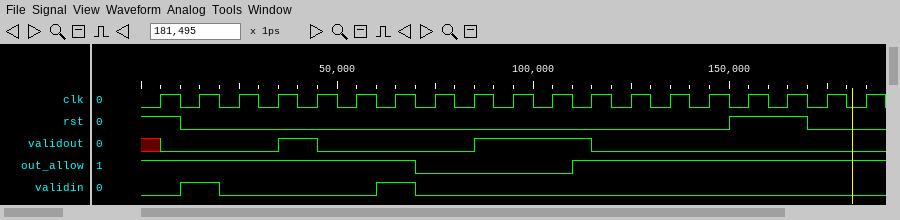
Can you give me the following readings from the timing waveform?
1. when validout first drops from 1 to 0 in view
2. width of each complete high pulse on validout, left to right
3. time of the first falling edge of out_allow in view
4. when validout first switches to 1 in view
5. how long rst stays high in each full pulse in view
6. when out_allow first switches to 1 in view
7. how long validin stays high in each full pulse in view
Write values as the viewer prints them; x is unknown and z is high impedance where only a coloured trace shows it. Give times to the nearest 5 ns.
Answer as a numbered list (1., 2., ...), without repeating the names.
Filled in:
1. 45 ns
2. 10 ns, 30 ns
3. 70 ns
4. 35 ns
5. 20 ns
6. 110 ns
7. 10 ns, 10 ns
